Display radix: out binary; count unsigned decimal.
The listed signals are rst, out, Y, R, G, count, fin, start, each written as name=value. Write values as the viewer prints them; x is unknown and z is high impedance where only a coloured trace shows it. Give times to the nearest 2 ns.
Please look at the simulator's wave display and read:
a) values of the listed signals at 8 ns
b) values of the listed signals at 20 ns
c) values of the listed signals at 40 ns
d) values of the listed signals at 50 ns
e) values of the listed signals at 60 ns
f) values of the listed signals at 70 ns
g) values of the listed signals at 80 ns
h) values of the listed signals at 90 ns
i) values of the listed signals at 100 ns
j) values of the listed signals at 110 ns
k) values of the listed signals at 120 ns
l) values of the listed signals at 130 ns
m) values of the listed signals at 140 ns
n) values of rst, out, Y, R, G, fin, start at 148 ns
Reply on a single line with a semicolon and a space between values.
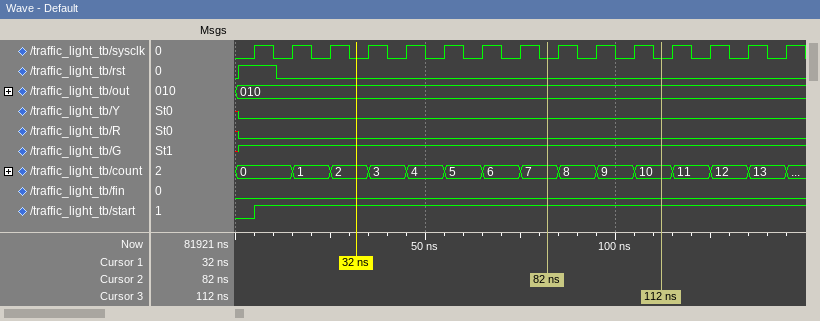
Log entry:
rst=1, out=010, Y=0, R=0, G=1, count=0, fin=0, start=1; rst=0, out=010, Y=0, R=0, G=1, count=1, fin=0, start=1; rst=0, out=010, Y=0, R=0, G=1, count=3, fin=0, start=1; rst=0, out=010, Y=0, R=0, G=1, count=4, fin=0, start=1; rst=0, out=010, Y=0, R=0, G=1, count=5, fin=0, start=1; rst=0, out=010, Y=0, R=0, G=1, count=6, fin=0, start=1; rst=0, out=010, Y=0, R=0, G=1, count=7, fin=0, start=1; rst=0, out=010, Y=0, R=0, G=1, count=8, fin=0, start=1; rst=0, out=010, Y=0, R=0, G=1, count=9, fin=0, start=1; rst=0, out=010, Y=0, R=0, G=1, count=10, fin=0, start=1; rst=0, out=010, Y=0, R=0, G=1, count=11, fin=0, start=1; rst=0, out=010, Y=0, R=0, G=1, count=12, fin=0, start=1; rst=0, out=010, Y=0, R=0, G=1, count=13, fin=0, start=1; rst=0, out=010, Y=0, R=0, G=1, fin=0, start=1
